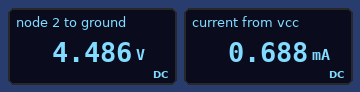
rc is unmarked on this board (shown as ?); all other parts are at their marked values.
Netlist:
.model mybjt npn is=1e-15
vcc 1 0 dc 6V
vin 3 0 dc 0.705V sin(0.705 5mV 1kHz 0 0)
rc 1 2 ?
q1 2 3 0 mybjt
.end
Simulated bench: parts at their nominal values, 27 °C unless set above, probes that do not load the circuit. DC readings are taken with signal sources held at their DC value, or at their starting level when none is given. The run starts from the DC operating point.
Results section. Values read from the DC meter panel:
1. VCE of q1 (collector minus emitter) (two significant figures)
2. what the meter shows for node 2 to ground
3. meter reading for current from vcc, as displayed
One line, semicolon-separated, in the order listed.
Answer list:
4.5 V; 4.486 V; 0.688 mA
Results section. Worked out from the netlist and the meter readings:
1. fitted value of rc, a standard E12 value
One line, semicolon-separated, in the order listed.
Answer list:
2.2 kΩ
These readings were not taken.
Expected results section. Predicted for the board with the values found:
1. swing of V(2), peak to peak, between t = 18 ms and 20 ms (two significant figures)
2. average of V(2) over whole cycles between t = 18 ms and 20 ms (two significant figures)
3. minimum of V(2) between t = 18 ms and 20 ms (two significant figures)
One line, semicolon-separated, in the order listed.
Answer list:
590 mV; 4.5 V; 4.2 V
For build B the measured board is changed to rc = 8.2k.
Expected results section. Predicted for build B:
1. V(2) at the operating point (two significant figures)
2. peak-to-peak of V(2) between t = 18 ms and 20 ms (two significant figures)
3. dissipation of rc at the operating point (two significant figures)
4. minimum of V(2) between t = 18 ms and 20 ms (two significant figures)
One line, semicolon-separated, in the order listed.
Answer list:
360 mV; 1.3 V; 3.9 mW; 70 mV
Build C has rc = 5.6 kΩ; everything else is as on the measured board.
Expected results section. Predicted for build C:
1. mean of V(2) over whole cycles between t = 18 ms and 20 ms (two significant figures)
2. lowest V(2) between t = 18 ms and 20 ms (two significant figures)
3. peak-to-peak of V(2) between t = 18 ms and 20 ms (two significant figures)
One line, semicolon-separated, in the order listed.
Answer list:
2.1 V; 1.3 V; 1.5 V
